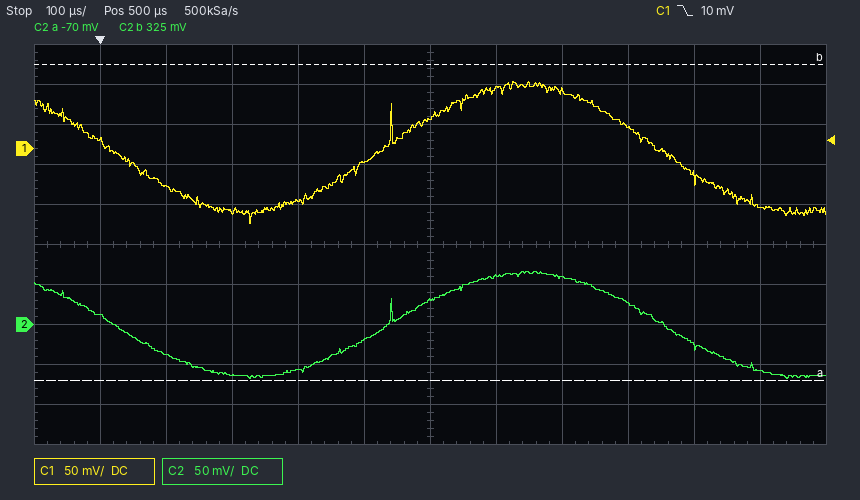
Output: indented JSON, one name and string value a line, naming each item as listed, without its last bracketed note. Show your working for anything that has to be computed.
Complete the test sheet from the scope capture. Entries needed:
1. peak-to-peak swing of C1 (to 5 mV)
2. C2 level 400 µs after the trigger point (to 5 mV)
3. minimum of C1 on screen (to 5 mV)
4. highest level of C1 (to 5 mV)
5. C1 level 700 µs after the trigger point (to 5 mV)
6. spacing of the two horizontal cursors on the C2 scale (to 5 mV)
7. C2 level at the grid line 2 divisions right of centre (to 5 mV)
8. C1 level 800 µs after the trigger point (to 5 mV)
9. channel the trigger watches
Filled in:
{
  "peak-to-peak swing of C1": "85 mV − (-95 mV) = 180 mV",
  "C2 level 400 µs after the trigger point": "-20 mV",
  "minimum of C1 on screen": "-95 mV",
  "highest level of C1": "85 mV",
  "C1 level 700 µs after the trigger point": "70 mV",
  "spacing of the two horizontal cursors on the C2 scale": "395 mV",
  "C2 level at the grid line 2 divisions right of centre": "60 mV",
  "C1 level 800 µs after the trigger point": "25 mV",
  "channel the trigger watches": "C1"
}
